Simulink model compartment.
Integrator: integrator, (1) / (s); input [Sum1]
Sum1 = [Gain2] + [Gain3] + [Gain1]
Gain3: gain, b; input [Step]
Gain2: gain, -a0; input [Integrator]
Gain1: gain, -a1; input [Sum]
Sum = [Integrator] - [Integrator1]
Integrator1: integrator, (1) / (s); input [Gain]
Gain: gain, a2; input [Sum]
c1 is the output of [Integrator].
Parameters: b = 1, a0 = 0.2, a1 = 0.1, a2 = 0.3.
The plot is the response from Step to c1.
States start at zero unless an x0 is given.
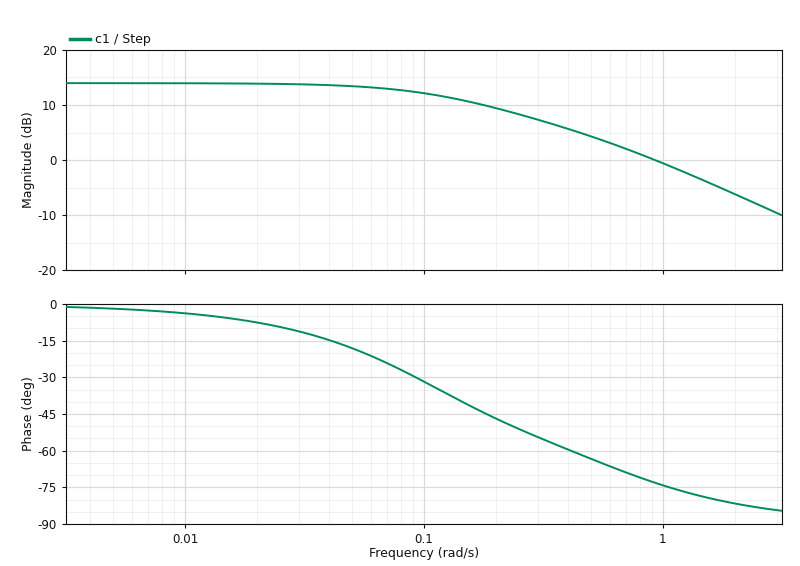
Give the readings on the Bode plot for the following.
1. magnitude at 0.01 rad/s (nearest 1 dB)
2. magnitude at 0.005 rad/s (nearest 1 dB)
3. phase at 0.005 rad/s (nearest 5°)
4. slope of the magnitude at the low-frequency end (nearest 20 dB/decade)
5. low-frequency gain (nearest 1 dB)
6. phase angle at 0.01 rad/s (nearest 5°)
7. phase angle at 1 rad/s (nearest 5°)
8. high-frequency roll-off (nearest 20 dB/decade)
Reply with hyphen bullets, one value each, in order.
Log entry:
- 14 dB
- 14 dB
- 0°
- 0 dB/decade
- 14 dB
- -5°
- -75°
- -20 dB/decade
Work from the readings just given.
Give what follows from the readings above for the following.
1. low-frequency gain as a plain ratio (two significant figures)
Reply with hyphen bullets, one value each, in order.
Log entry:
- 5.0
